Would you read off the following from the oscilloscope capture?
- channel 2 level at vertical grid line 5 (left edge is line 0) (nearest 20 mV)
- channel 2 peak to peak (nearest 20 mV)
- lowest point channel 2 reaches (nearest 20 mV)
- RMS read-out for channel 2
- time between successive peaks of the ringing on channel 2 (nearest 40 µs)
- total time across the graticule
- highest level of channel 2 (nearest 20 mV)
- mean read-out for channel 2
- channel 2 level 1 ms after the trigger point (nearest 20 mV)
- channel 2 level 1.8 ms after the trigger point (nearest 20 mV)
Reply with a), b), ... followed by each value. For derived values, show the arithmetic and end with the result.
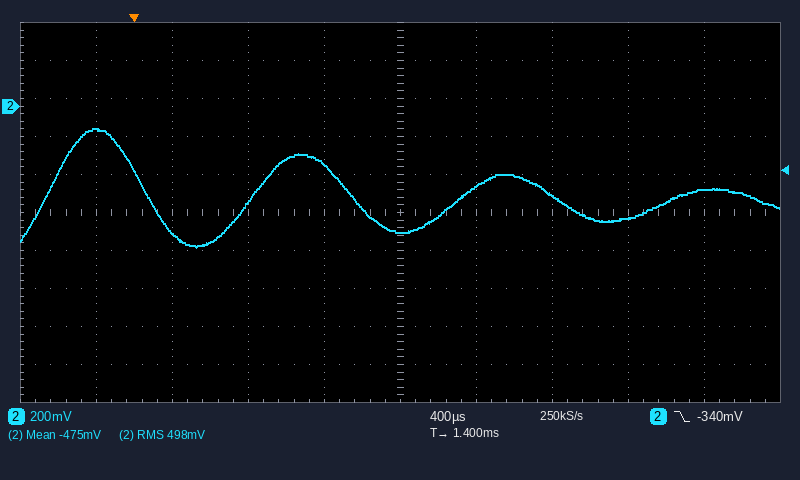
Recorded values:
a) -660 mV
b) -120 mV − (-740 mV) = 620 mV
c) -740 mV
d) 498 mV
e) 1.08 ms
f) 4 ms
g) -120 mV
h) -475 mV
i) -300 mV
j) -420 mV
